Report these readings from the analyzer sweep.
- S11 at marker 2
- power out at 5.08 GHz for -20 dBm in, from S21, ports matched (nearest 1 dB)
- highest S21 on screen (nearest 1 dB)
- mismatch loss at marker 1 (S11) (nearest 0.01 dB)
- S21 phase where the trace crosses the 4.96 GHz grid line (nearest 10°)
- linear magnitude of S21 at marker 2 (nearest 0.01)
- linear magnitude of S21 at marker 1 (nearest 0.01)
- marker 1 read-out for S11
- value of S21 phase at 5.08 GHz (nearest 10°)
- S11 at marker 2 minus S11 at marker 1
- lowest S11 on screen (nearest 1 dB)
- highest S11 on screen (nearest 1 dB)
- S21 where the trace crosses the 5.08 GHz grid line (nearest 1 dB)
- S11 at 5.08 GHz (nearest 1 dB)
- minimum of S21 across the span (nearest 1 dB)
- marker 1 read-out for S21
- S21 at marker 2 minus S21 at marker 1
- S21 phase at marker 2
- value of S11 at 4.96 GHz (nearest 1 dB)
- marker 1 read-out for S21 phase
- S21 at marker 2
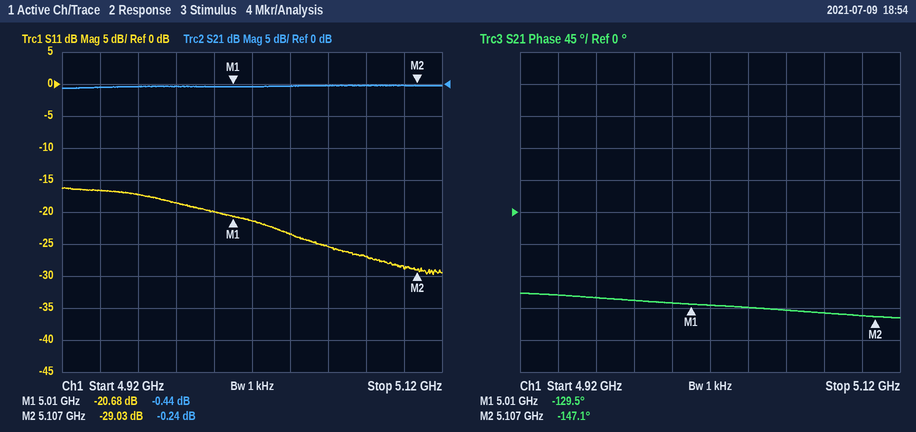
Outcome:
-29.03 dB
-20 dBm
0 dB
0.04 dB
-120°
0.97
0.95
-20.68 dB
-140°
-8.35 dB
-30 dB
-16 dB
0 dB
-27 dB
-1 dB
-0.44 dB
0.20 dB
-147.1°
-17 dB
-129.5°
-0.24 dB
